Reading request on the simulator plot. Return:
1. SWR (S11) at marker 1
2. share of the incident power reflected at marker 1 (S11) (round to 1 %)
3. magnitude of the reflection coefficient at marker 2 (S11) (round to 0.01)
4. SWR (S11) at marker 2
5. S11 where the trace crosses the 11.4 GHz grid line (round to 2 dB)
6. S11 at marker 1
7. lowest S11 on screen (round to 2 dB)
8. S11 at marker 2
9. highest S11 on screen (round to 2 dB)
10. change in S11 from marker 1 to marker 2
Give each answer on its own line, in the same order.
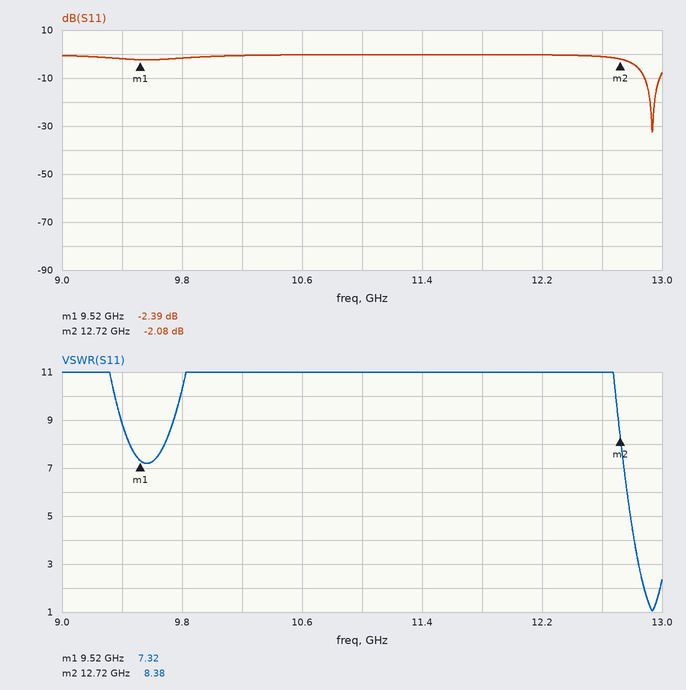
7.32
58 %
0.79
8.38
0 dB
-2.39 dB
-32 dB
-2.08 dB
0 dB
0.31 dB
